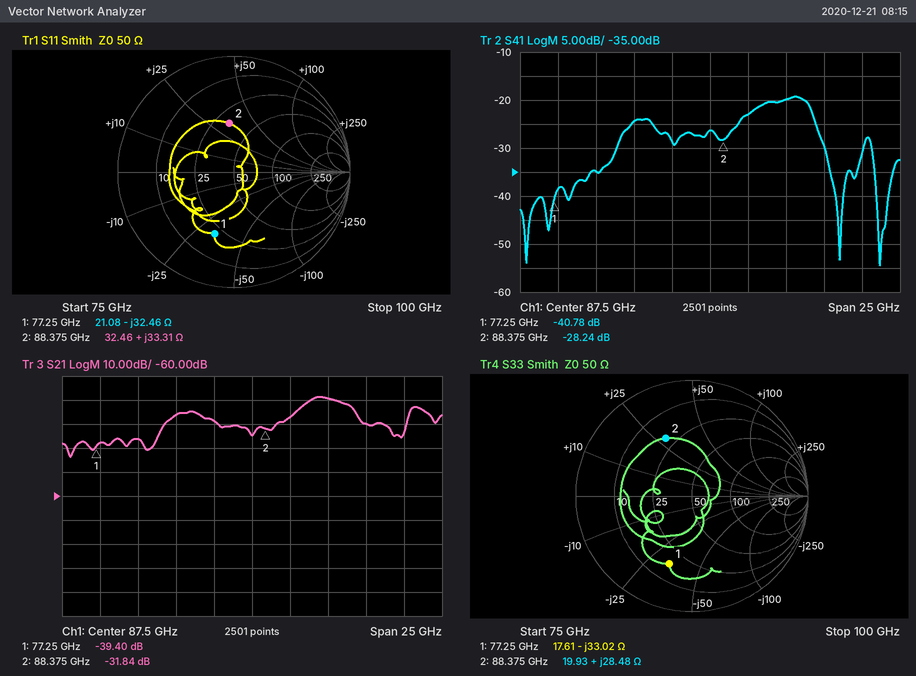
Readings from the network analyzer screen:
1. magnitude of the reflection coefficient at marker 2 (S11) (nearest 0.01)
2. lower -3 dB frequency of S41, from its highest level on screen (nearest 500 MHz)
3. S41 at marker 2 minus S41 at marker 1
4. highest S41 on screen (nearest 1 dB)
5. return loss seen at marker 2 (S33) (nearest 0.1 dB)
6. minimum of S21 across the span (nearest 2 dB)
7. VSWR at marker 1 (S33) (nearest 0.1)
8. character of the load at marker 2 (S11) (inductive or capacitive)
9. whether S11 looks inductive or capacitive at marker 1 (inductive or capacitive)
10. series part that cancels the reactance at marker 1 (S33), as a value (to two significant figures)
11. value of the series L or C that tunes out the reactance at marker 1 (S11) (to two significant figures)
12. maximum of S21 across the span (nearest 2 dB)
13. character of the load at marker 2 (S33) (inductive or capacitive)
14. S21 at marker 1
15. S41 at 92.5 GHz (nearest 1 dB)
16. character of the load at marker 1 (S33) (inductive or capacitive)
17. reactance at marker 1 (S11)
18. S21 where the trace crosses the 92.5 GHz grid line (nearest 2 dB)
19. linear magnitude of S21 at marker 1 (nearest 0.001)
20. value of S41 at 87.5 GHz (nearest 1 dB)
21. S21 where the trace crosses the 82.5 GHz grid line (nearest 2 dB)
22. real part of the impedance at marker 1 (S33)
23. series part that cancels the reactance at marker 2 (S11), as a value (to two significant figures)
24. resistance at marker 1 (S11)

0.42
90.5 GHz
12.54 dB
-19 dB
5.2 dB
-44 dB
4.2
inductive
capacitive
68 pH
67 pH
-18 dB
inductive
-39.40 dB
-20 dB
capacitive
-32.46 Ω
-20 dB
0.011
-26 dB
-26 dB
17.61 Ω
54 fF
21.08 Ω
